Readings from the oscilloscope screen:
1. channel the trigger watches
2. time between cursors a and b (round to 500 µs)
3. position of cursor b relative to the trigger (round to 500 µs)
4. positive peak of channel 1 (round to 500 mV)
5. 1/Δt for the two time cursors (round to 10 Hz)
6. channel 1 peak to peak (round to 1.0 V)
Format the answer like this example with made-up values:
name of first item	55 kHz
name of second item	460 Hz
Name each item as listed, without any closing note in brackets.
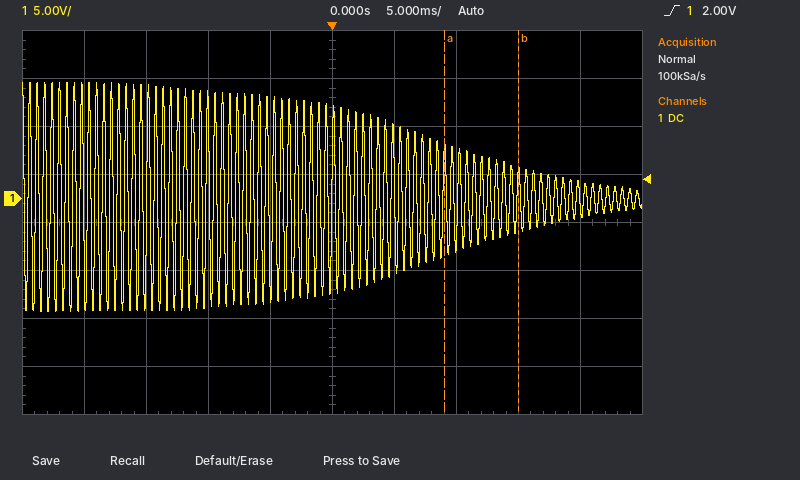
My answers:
channel the trigger watches	channel 1
time between cursors a and b	6.0 ms
position of cursor b relative to the trigger	+15.0 ms
positive peak of channel 1	12.0 V
1/Δt for the two time cursors	170 Hz
channel 1 peak to peak	24.0 V
